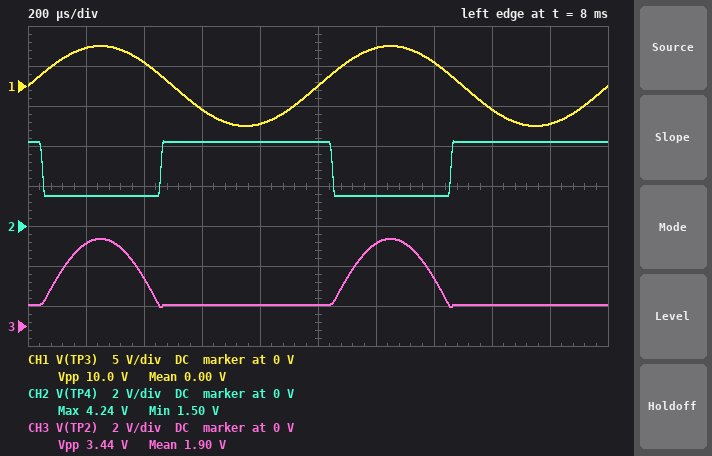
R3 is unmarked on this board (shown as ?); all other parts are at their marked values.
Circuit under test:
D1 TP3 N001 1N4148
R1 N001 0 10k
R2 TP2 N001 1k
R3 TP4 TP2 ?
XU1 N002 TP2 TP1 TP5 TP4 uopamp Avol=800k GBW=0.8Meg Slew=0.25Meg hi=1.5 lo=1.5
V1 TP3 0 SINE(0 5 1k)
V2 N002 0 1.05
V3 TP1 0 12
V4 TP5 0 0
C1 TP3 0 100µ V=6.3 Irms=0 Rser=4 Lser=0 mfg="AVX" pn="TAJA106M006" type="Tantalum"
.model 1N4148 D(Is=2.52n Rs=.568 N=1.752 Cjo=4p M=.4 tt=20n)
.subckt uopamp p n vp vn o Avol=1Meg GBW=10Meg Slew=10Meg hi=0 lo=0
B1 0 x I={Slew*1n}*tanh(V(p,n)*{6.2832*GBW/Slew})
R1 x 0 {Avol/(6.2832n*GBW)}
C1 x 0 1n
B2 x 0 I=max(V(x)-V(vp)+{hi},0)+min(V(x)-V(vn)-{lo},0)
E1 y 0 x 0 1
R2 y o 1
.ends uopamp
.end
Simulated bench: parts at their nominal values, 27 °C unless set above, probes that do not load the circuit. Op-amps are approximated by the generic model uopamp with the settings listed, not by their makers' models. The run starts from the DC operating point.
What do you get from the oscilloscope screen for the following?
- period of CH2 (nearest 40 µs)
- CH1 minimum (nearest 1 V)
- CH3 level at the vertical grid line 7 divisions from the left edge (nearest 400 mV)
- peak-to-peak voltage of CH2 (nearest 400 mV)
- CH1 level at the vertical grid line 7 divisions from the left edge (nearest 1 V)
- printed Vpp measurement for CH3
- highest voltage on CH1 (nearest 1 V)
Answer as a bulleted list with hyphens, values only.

- 1.00 ms
- -5 V
- 2.4 V
- 2.8 V
- 3 V
- 3.44 V
- 5 V
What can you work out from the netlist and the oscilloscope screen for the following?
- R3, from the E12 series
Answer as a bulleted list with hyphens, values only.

- 33 kΩ
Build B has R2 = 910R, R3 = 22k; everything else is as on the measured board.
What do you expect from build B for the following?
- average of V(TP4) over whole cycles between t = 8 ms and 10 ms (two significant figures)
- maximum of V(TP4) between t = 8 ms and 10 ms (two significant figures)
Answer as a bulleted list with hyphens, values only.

- 2.5 V
- 3.2 V
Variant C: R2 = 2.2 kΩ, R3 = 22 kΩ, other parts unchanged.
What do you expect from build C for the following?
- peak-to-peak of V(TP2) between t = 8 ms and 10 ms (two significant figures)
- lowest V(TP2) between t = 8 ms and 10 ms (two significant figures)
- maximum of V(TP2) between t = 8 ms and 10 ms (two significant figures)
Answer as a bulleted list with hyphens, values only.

- 3.2 V
- 1.0 V
- 4.2 V
